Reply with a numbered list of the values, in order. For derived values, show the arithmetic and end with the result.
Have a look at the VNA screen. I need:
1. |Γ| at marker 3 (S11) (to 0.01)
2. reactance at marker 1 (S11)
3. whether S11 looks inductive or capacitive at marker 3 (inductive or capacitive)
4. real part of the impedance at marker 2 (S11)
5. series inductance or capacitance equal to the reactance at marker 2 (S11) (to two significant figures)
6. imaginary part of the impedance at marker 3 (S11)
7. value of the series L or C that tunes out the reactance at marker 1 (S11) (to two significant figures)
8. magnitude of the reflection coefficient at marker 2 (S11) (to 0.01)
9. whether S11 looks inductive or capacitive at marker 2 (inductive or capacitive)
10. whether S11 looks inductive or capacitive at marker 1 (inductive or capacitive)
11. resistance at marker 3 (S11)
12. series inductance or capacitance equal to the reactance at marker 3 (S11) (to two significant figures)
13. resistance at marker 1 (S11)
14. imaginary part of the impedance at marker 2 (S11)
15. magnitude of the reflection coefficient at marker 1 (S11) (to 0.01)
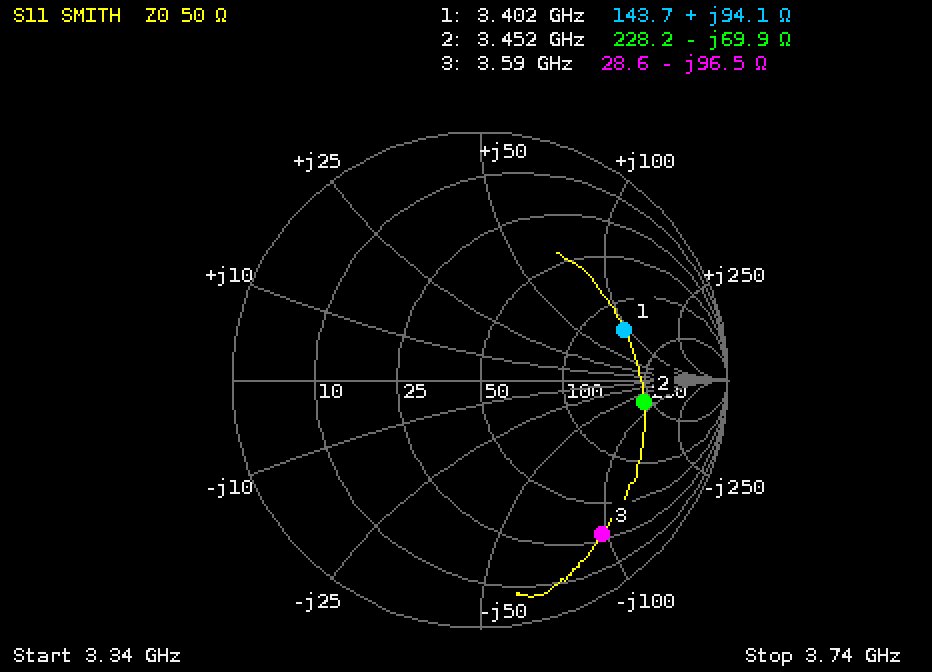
1. 0.79
2. +94.1 Ω
3. capacitive
4. 228.2 Ω
5. C = 1/(2π × 3.452 GHz × 69.9 Ω) ≈ 660 fF
6. -96.5 Ω
7. C = 1/(2π × 3.402 GHz × 94.1 Ω) ≈ 497 fF, so 500 fF to two significant figures
8. 0.67
9. capacitive
10. inductive
11. 28.6 Ω
12. C = 1/(2π × 3.59 GHz × 96.5 Ω) ≈ 459 fF, so 460 fF to two significant figures
13. 143.7 Ω
14. -69.9 Ω
15. 0.62
